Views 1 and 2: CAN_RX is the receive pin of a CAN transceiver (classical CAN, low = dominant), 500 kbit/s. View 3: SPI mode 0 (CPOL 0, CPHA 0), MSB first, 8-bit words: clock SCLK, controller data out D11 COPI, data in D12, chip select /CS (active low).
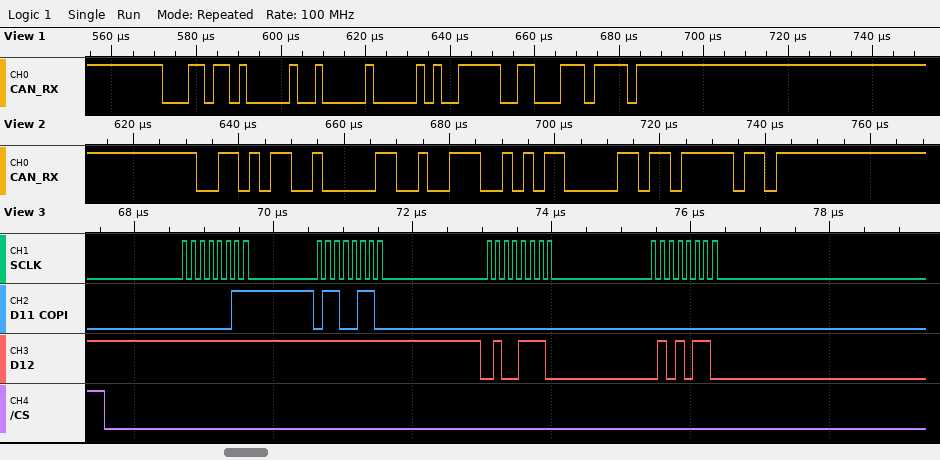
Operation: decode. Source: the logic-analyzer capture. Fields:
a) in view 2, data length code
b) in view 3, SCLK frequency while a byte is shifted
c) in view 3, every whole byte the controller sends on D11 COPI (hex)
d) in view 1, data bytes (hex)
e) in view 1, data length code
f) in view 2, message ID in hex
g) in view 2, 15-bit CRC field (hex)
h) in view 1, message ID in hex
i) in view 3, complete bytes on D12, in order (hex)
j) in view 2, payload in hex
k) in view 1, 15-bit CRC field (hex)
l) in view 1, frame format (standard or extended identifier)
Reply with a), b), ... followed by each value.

a) 2
b) 8 MHz
c) 03 66 00 00
d) 00 27
e) 2
f) 0x359
g) 0x05BF
h) 0x1B4
i) FF FF 4E 56
j) 4E 56
k) 0x6C77
l) standard
